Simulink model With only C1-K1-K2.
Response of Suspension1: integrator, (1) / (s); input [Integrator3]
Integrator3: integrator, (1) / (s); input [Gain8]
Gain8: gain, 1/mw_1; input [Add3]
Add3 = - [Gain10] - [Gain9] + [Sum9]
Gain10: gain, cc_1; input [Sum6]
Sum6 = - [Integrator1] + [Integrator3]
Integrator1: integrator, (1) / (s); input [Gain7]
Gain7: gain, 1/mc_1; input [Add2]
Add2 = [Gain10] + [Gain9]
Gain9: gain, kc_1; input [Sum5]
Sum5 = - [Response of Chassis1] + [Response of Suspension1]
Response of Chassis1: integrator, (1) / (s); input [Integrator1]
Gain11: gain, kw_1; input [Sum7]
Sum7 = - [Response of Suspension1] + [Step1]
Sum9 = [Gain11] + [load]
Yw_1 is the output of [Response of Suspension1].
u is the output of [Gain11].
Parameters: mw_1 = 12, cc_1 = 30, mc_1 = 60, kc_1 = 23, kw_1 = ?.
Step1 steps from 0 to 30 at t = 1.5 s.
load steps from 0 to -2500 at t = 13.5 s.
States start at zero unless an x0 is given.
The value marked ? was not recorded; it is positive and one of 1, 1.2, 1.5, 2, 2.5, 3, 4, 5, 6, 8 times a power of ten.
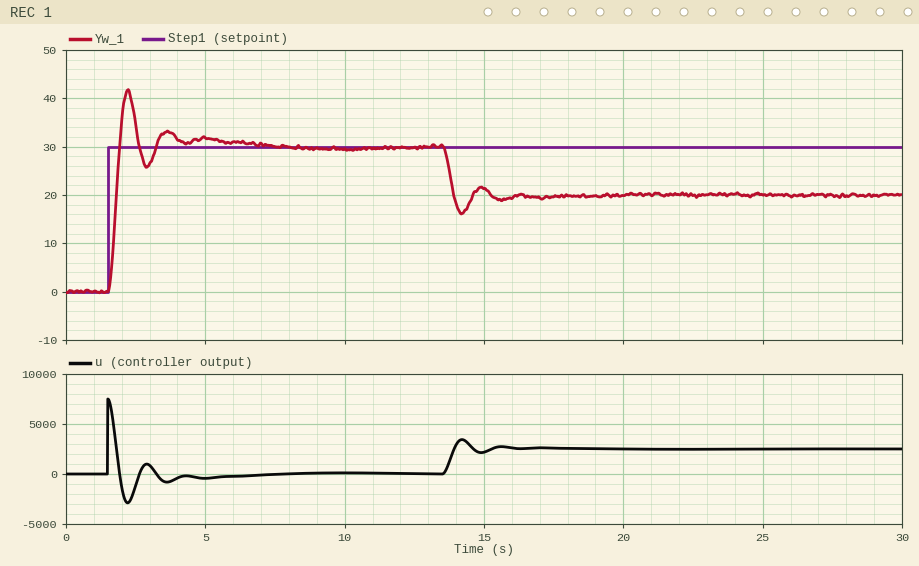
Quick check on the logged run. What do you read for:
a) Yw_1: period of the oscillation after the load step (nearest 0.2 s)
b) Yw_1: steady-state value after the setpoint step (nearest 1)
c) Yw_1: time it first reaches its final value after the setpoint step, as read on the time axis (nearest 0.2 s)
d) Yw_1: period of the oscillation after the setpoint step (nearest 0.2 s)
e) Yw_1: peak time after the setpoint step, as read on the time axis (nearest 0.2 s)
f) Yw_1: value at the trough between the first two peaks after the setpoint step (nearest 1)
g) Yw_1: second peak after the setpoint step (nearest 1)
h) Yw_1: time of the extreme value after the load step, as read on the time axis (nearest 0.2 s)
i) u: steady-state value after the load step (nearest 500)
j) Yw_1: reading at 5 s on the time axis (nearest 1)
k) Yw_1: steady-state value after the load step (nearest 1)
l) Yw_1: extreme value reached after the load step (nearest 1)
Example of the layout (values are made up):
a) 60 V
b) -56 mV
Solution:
a) 1.4 s
b) 30
c) 2.0 s
d) 1.4 s
e) 2.2 s
f) 26
g) 33
h) 14.2 s
i) 2500
j) 32
k) 20
l) 16
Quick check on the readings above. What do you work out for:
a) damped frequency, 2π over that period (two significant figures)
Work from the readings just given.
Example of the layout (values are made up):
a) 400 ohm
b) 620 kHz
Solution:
a) 4.5 rad/s
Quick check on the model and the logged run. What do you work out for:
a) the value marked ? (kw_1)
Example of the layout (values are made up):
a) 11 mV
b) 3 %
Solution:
a) 250
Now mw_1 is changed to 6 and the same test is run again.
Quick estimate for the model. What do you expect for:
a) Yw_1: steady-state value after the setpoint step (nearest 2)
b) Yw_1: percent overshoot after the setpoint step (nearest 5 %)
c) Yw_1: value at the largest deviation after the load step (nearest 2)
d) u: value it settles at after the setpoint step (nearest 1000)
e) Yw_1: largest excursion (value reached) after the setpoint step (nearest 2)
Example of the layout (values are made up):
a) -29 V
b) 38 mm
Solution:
a) 30
b) 25 %
c) 18
d) 0
e) 38
